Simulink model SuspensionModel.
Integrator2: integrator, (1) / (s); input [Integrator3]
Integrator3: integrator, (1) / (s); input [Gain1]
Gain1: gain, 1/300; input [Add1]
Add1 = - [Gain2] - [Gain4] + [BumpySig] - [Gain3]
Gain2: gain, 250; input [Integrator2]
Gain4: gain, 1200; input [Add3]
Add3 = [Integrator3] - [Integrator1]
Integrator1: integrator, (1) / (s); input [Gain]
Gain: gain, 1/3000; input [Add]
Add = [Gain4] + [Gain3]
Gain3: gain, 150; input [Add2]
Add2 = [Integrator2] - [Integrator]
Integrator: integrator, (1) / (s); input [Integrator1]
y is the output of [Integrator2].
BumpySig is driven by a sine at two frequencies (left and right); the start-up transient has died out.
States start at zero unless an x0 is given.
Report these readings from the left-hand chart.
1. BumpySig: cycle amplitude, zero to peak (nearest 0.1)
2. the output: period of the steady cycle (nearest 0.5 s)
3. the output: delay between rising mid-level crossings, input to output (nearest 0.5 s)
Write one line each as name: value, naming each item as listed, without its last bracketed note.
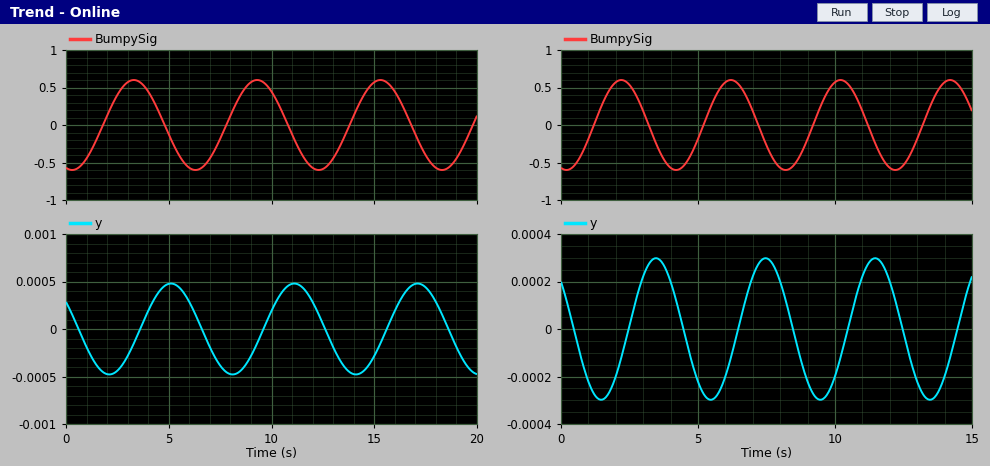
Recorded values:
BumpySig: cycle amplitude, zero to peak: 0.6
the output: period of the steady cycle: 6.0 s
the output: delay between rising mid-level crossings, input to output: 2.0 s
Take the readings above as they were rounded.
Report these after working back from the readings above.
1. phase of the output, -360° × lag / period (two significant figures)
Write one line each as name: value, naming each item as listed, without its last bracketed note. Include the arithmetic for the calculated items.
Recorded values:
phase of the output, -360° × lag / period: -360 × 2 / 6 = -120°
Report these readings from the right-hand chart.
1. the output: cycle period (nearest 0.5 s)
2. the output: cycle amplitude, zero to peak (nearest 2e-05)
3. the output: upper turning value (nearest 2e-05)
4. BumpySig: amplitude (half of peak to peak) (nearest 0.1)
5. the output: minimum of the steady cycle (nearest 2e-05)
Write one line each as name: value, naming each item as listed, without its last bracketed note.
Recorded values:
the output: cycle period: 4.0 s
the output: cycle amplitude, zero to peak: 0.00030
the output: upper turning value: 0.00030
BumpySig: amplitude (half of peak to peak): 0.6
the output: minimum of the steady cycle: -0.00030
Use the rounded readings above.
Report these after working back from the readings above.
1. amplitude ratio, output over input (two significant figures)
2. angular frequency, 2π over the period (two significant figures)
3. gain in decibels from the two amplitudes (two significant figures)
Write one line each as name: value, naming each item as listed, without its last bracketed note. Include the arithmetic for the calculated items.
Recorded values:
amplitude ratio, output over input: 0.0003 / 0.6 = 0.00050
angular frequency, 2π over the period: 2π / 4 = 1.6 rad/s
gain in decibels from the two amplitudes: 20 log10(0.0003 / 0.6) = -66 dB
